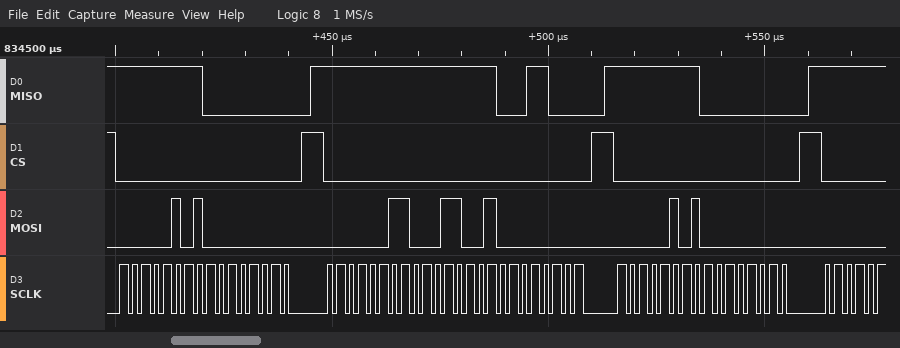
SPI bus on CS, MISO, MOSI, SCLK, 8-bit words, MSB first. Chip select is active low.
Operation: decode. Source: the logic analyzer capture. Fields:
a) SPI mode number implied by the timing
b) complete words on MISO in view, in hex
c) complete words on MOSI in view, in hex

0
FF, 00, FF, FF, 18, FF, 00
05, 00, 03, 19, 00, 05, 00
